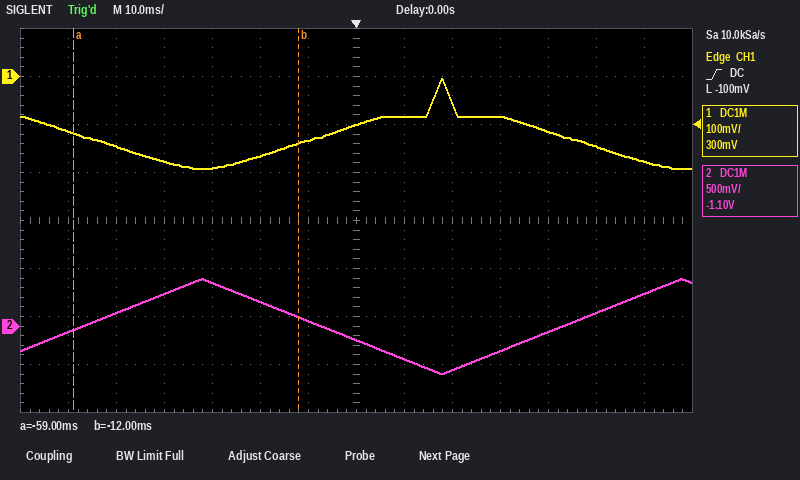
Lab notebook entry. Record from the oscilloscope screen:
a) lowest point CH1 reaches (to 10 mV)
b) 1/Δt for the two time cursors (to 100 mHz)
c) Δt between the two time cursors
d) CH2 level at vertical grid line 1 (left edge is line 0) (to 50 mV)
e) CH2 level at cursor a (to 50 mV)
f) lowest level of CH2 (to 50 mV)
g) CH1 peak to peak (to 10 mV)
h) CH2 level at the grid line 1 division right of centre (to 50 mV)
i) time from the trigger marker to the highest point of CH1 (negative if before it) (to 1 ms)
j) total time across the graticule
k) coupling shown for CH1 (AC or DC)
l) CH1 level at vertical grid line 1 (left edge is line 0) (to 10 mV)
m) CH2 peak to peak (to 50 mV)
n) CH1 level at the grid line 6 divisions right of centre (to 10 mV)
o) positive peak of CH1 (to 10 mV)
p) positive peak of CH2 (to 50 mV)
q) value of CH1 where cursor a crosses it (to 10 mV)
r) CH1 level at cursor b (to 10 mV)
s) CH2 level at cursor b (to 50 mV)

-190 mV
21.3 Hz
47 ms
-50 mV
-50 mV
-500 mV
190 mV
-350 mV
+18 ms
140 ms
DC
-110 mV
1.00 V
-180 mV
0 mV
500 mV
-120 mV
-140 mV
100 mV
